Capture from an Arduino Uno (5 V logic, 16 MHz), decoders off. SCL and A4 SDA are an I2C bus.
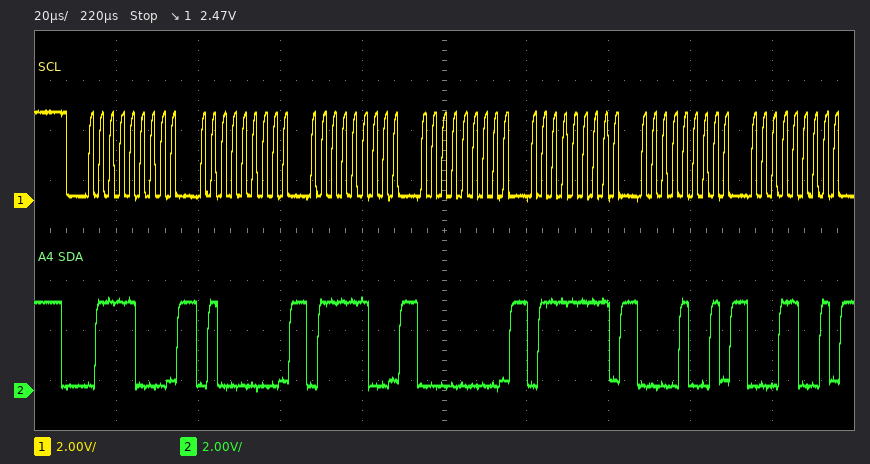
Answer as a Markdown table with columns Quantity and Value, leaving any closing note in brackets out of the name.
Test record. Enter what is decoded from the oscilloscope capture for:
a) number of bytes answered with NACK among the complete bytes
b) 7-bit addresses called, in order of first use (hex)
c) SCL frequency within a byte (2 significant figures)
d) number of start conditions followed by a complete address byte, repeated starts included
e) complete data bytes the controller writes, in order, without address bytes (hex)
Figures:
| Quantity | Value |
|---|---|
| number of bytes answered with NACK among the complete bytes | 0 |
| 7-bit addresses called, in order of first use | 0x3C |
| SCL frequency within a byte | 400 kHz |
| number of start conditions followed by a complete address byte, repeated starts included | 1 |
| complete data bytes the controller writes, in order, without address bytes | 40 7C 00 7F 09 19 |
